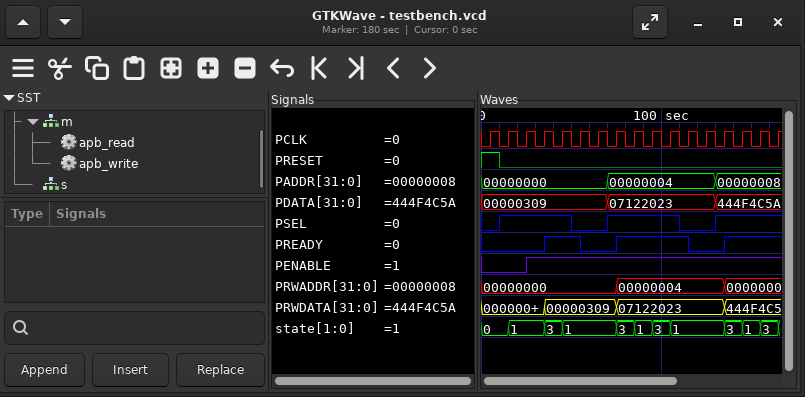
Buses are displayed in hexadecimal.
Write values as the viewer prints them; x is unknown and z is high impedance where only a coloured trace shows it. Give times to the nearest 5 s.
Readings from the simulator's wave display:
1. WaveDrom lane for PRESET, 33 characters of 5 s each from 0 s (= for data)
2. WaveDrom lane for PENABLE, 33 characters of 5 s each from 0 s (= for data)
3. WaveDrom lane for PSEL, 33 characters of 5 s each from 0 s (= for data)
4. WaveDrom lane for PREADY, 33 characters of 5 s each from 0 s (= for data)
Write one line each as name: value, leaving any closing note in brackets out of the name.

WaveDrom lane for PRESET, 33 characters of 5 s each from 0 s: {name: 'PRESET', wave: '1.0..............................'}
WaveDrom lane for PENABLE, 33 characters of 5 s each from 0 s: {name: 'PENABLE', wave: '0....1...........................'}
WaveDrom lane for PSEL, 33 characters of 5 s each from 0 s: {name: 'PSEL', wave: '0.1.......0...1.......0...1......'}
WaveDrom lane for PREADY, 33 characters of 5 s each from 0 s: {name: 'PREADY', wave: '0......1...0...1.......0...1.....'}
